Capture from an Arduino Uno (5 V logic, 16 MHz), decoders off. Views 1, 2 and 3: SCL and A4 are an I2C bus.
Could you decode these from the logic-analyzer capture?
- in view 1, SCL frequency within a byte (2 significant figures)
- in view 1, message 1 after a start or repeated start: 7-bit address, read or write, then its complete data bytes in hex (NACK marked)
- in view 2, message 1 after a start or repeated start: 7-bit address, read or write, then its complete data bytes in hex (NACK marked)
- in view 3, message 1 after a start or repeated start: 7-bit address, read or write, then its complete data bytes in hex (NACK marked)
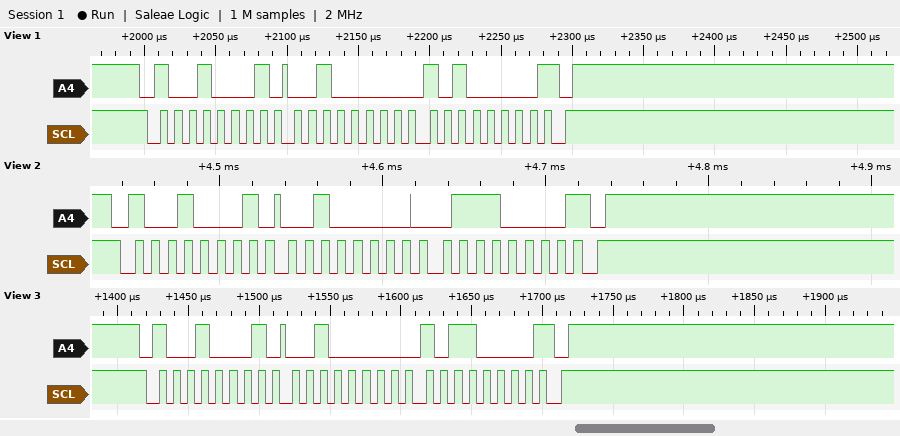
100 kHz
0x48 read: 20 A0 NACK
0x48 read: 20 70 NACK
0x48 read: 20 B0 NACK
